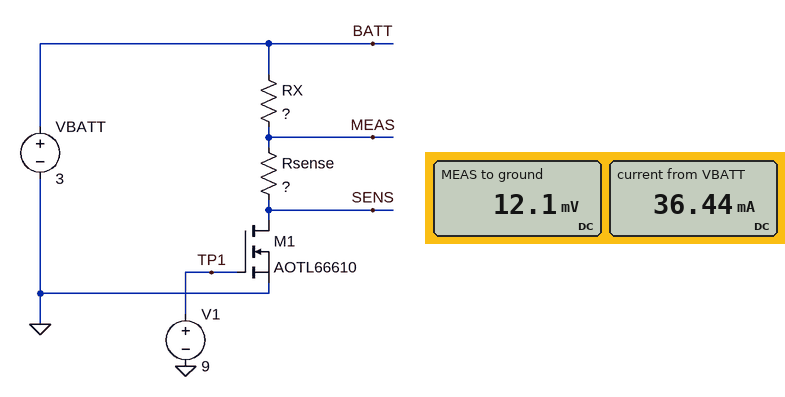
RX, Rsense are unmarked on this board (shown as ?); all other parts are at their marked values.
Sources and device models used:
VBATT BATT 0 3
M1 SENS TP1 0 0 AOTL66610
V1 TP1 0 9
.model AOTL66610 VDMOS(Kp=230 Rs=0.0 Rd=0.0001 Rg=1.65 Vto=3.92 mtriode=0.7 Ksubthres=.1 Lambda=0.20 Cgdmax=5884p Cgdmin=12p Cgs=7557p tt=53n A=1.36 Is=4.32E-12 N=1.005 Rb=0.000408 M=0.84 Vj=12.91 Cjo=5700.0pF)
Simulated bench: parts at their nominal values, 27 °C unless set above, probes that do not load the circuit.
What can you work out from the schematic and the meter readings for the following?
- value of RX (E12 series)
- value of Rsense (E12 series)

82 Ω
0.33 Ω
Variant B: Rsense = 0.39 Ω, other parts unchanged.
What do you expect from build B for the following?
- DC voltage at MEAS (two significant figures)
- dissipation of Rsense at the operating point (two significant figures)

14 mV
520 µW
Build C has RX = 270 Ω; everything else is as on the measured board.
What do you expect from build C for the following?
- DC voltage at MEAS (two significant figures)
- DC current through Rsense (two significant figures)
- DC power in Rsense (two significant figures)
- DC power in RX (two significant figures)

3.7 mV
11 mA
41 µW
33 mW
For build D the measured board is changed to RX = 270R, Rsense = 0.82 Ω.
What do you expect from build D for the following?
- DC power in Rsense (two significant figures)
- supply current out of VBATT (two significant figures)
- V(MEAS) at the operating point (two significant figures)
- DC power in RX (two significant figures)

100 µW
11 mA
9.1 mV
33 mW
